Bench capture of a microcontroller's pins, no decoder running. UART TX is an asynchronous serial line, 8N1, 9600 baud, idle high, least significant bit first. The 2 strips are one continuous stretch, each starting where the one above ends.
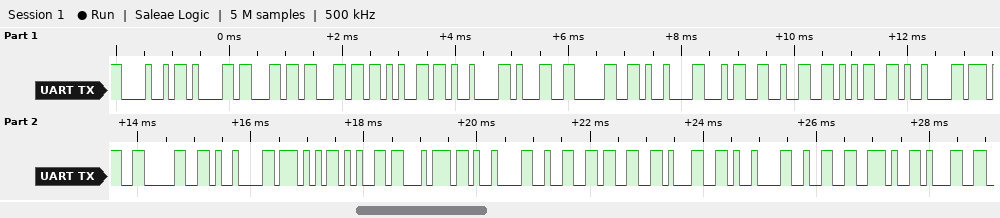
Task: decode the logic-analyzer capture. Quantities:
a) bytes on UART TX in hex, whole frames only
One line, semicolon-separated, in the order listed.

48 61 6C 6C 65 09 31 30 09 34 32 35 09 37 30 09 57 65 74 09 32 33 31 09 32 2E 31
